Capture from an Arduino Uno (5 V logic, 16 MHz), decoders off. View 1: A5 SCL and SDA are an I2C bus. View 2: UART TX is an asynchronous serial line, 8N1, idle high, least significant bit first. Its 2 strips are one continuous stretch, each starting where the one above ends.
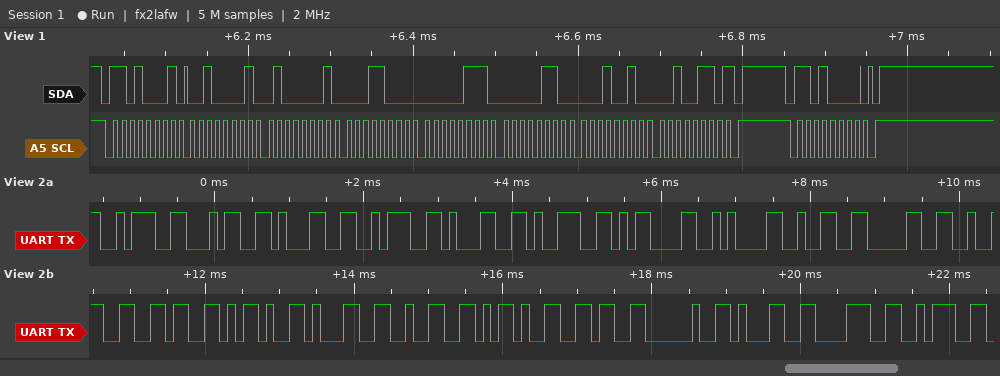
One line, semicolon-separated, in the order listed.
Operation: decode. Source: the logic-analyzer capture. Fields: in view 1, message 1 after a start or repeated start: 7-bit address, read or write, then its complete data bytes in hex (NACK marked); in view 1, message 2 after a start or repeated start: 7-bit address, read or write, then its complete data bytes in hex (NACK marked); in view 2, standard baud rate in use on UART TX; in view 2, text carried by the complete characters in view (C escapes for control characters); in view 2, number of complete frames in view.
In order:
0x68 read: 21 41 18 07 06 12 26 NACK; 0x68 write; 9600 baud; ":41:19\r\n2026-12-6 18:"; 21
